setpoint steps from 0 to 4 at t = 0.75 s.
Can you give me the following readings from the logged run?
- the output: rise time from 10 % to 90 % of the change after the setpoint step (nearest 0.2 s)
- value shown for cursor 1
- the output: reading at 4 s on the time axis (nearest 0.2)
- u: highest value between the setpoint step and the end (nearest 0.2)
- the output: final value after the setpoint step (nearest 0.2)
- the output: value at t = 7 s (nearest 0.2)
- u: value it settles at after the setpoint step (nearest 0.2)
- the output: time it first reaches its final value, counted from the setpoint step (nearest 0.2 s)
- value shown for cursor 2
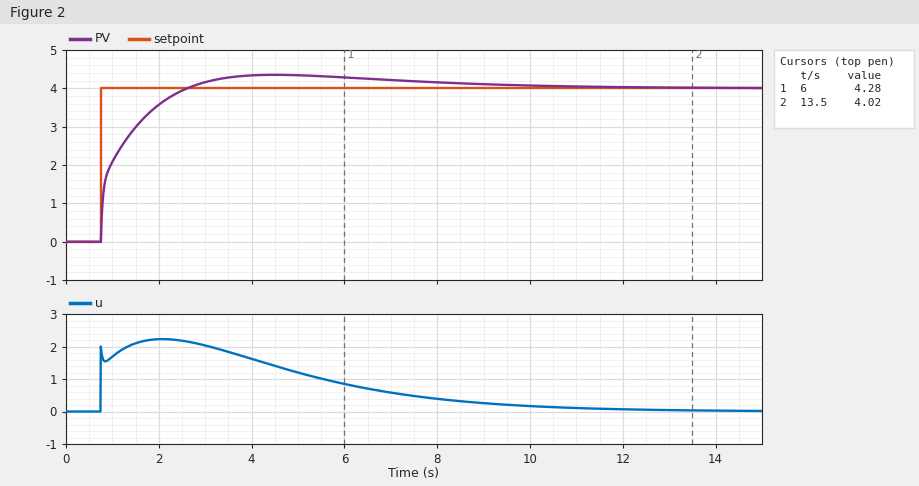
1.2 s
4.28
4.4
2.2
4.0
4.2
0.0
1.8 s
4.02
